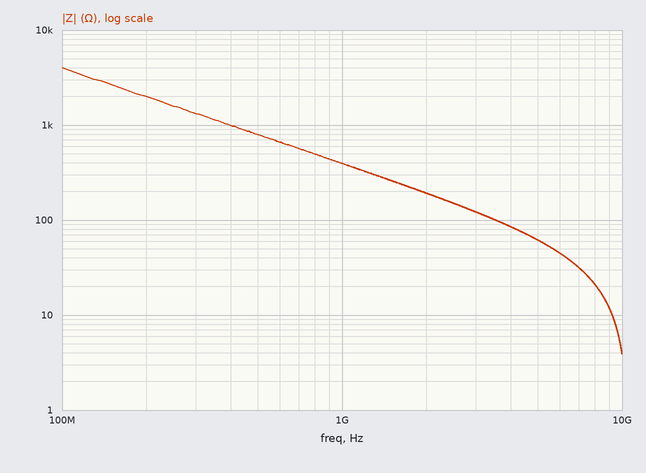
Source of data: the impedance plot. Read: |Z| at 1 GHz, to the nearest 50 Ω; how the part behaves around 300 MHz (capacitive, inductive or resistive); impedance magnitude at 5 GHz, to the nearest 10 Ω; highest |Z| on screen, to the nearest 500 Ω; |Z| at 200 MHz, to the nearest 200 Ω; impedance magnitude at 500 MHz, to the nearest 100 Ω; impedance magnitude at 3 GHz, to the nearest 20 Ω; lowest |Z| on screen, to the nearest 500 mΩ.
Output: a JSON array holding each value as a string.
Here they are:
["400 Ω", "capacitive", "60 Ω", "4.0 kΩ", "2.0 kΩ", "800 Ω", "120 Ω", "4.0 Ω"]
